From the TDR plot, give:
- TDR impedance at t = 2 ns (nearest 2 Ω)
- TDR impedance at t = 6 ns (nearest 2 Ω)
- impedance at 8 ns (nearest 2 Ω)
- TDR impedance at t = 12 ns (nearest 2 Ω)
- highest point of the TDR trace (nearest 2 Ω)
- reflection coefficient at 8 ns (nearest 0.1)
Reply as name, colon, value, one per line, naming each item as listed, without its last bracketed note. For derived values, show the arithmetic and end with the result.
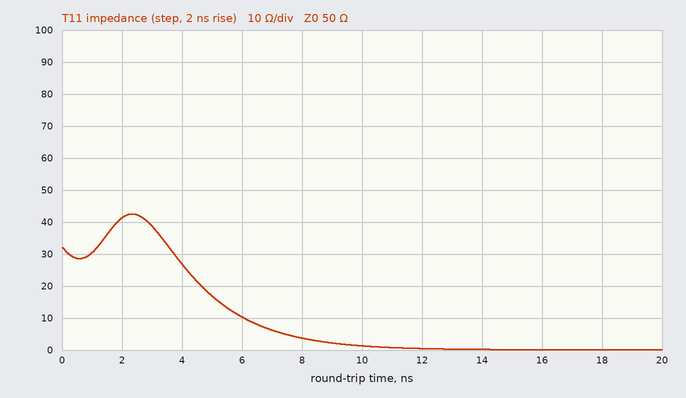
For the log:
TDR impedance at t = 2 ns: 42 Ω
TDR impedance at t = 6 ns: 10 Ω
impedance at 8 ns: 4 Ω
TDR impedance at t = 12 ns: 0 Ω
highest point of the TDR trace: 42 Ω
reflection coefficient at 8 ns: (4 − 50)/(4 + 50) ≈ -0.9
